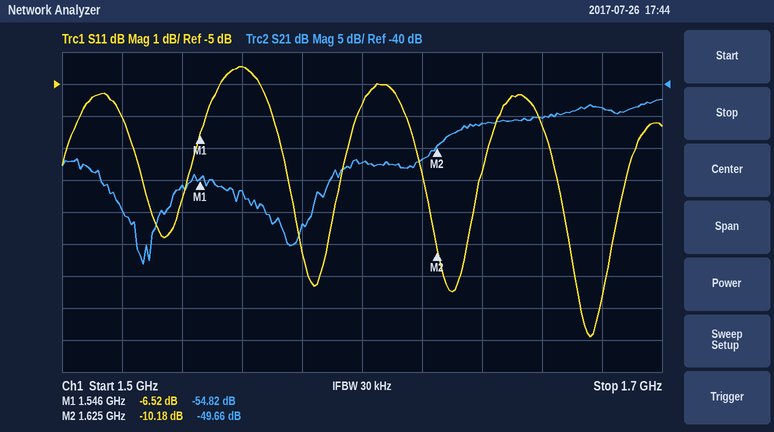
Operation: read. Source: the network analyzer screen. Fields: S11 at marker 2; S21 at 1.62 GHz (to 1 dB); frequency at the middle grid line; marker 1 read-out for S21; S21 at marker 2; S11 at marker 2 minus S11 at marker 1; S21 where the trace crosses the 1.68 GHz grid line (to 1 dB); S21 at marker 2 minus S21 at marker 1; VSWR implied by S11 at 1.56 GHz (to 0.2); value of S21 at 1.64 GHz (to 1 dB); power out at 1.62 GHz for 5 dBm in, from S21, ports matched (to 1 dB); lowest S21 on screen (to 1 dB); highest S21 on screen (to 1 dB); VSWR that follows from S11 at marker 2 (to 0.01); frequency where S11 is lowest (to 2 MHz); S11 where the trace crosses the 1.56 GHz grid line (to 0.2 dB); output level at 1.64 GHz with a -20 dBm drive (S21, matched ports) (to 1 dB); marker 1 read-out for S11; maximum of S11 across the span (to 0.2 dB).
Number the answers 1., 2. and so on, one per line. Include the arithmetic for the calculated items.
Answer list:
1. -10.18 dB
2. -52 dB
3. 1.6 GHz
4. -54.82 dB
5. -49.66 dB
6. -10.18 − (-6.52) = -3.66 dB
7. -44 dB
8. -49.66 − (-54.82) = 5.16 dB
9. |Γ| = 10^(-4.4/20) = 0.6026; VSWR = (1 + 0.6026)/(1 − 0.6026) ≈ 4.0
10. -46 dB
11. 5 dBm + (-52 dB) = -47 dBm
12. -68 dB
13. -42 dB
14. (1 + 0.3097)/(1 − 0.3097) ≈ 1.90
15. 1.676 GHz
16. -4.4 dB
17. -20 dBm + (-46 dB) = -66 dBm
18. -6.52 dB
19. -4.4 dB
